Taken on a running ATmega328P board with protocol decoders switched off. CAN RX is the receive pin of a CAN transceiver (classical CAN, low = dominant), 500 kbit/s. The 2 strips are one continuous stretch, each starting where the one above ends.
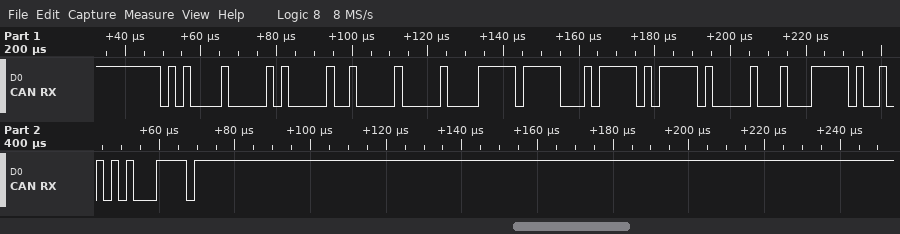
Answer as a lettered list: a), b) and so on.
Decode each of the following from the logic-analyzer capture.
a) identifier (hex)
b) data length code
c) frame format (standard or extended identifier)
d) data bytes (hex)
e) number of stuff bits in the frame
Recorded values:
a) 0x508
b) 8
c) standard
d) 08 00 1F F9 7E FC 02 3F
e) 10
